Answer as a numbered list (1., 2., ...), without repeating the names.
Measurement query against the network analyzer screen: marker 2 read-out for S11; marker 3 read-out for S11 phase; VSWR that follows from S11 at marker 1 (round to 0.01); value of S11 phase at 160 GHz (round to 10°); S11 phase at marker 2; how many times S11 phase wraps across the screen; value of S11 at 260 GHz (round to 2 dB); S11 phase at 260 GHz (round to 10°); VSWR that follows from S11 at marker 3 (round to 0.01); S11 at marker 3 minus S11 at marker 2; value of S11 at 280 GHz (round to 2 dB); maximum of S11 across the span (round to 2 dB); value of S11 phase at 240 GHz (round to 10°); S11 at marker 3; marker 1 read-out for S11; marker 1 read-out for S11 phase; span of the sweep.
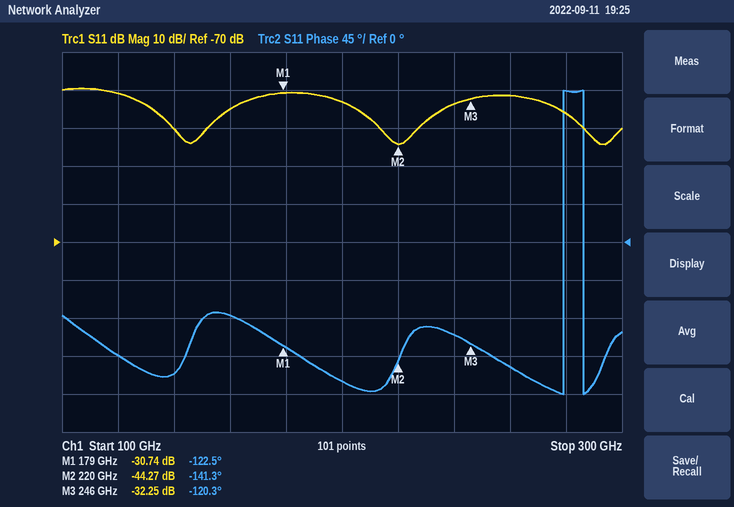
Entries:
1. -44.27 dB
2. -120.3°
3. 1.06
4. -90°
5. -141.3°
6. 2
7. -32 dB
8. -150°
9. 1.05
10. 12.02 dB
11. -36 dB
12. -30 dB
13. -110°
14. -32.25 dB
15. -30.74 dB
16. -122.5°
17. 200 GHz
